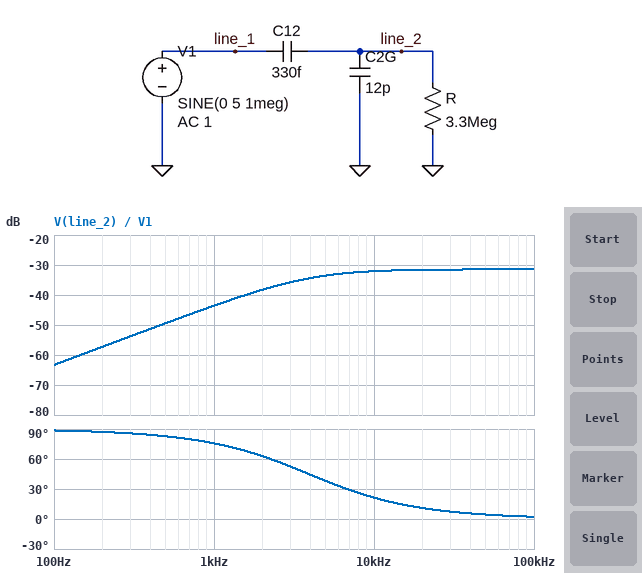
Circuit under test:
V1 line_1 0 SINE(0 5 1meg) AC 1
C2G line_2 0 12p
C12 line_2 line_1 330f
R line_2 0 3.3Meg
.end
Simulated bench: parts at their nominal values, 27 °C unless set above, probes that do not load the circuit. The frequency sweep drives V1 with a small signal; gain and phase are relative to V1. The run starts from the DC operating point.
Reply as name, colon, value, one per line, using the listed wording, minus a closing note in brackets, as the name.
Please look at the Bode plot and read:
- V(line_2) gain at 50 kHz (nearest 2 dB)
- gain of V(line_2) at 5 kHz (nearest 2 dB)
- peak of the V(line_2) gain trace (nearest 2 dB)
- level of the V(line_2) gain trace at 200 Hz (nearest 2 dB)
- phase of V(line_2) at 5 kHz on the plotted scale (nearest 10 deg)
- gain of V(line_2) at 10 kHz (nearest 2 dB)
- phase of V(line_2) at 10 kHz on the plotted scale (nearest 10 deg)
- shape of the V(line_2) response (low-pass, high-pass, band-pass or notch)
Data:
V(line_2) gain at 50 kHz: -32 dB
gain of V(line_2) at 5 kHz: -34 dB
peak of the V(line_2) gain trace: -32 dB
level of the V(line_2) gain trace at 200 Hz: -58 dB
phase of V(line_2) at 5 kHz on the plotted scale: 40 deg
gain of V(line_2) at 10 kHz: -32 dB
phase of V(line_2) at 10 kHz on the plotted scale: 20 deg
shape of the V(line_2) response: high-pass
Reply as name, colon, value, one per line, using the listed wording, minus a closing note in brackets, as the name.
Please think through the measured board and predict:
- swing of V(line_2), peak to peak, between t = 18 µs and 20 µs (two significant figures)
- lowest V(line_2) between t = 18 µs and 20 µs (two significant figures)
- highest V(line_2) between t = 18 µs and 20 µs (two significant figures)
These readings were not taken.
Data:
swing of V(line_2), peak to peak, between t = 18 µs and 20 µs: 270 mV
lowest V(line_2) between t = 18 µs and 20 µs: -130 mV
highest V(line_2) between t = 18 µs and 20 µs: 130 mV
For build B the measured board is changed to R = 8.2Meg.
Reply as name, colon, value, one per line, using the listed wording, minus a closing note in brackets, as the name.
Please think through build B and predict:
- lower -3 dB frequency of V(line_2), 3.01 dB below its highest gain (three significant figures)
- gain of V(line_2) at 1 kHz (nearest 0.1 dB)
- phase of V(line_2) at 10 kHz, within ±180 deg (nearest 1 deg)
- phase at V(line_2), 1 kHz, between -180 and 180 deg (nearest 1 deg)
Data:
lower -3 dB frequency of V(line_2), 3.01 dB below its highest gain: 1.57 kHz
gain of V(line_2) at 1 kHz: -36.9 dB
phase of V(line_2) at 10 kHz, within ±180 deg: 9 deg
phase at V(line_2), 1 kHz, between -180 and 180 deg: 58 deg
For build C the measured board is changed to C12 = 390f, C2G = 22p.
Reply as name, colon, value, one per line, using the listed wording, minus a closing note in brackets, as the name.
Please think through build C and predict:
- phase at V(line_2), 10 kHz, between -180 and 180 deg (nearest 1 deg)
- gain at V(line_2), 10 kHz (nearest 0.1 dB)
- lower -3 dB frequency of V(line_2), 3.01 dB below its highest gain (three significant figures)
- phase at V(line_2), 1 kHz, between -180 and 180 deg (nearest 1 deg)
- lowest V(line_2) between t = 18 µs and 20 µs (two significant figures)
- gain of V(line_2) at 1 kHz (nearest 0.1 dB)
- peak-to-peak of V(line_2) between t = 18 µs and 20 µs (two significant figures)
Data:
phase at V(line_2), 10 kHz, between -180 and 180 deg: 12 deg
gain at V(line_2), 10 kHz: -35.4 dB
lower -3 dB frequency of V(line_2), 3.01 dB below its highest gain: 2.15 kHz
phase at V(line_2), 1 kHz, between -180 and 180 deg: 65 deg
lowest V(line_2) between t = 18 µs and 20 µs: -87 mV
gain of V(line_2) at 1 kHz: -42.7 dB
peak-to-peak of V(line_2) between t = 18 µs and 20 µs: 170 mV
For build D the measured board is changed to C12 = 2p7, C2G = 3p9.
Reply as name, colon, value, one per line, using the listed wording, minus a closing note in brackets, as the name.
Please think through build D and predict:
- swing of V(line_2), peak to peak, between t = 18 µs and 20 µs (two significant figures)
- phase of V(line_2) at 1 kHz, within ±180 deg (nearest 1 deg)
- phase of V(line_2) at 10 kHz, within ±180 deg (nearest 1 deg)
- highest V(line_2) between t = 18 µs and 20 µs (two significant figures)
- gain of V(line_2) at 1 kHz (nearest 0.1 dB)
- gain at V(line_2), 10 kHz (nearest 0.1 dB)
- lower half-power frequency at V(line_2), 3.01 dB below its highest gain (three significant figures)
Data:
swing of V(line_2), peak to peak, between t = 18 µs and 20 µs: 4.1 V
phase of V(line_2) at 1 kHz, within ±180 deg: 82 deg
phase of V(line_2) at 10 kHz, within ±180 deg: 36 deg
highest V(line_2) between t = 18 µs and 20 µs: 2.0 V
gain of V(line_2) at 1 kHz: -25.1 dB
gain at V(line_2), 10 kHz: -9.6 dB
lower half-power frequency at V(line_2), 3.01 dB below its highest gain: 7.31 kHz
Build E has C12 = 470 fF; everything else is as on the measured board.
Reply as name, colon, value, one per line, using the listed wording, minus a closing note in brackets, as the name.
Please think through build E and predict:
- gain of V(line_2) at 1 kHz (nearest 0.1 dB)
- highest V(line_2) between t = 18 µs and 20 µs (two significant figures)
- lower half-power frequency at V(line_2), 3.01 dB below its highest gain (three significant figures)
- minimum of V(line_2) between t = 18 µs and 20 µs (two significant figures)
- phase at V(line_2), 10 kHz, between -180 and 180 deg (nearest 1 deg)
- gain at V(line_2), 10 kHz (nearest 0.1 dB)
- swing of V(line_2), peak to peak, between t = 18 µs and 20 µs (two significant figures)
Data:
gain of V(line_2) at 1 kHz: -40.5 dB
highest V(line_2) between t = 18 µs and 20 µs: 190 mV
lower half-power frequency at V(line_2), 3.01 dB below its highest gain: 3.87 kHz
minimum of V(line_2) between t = 18 µs and 20 µs: -190 mV
phase at V(line_2), 10 kHz, between -180 and 180 deg: 21 deg
gain at V(line_2), 10 kHz: -29.1 dB
swing of V(line_2), peak to peak, between t = 18 µs and 20 µs: 380 mV
